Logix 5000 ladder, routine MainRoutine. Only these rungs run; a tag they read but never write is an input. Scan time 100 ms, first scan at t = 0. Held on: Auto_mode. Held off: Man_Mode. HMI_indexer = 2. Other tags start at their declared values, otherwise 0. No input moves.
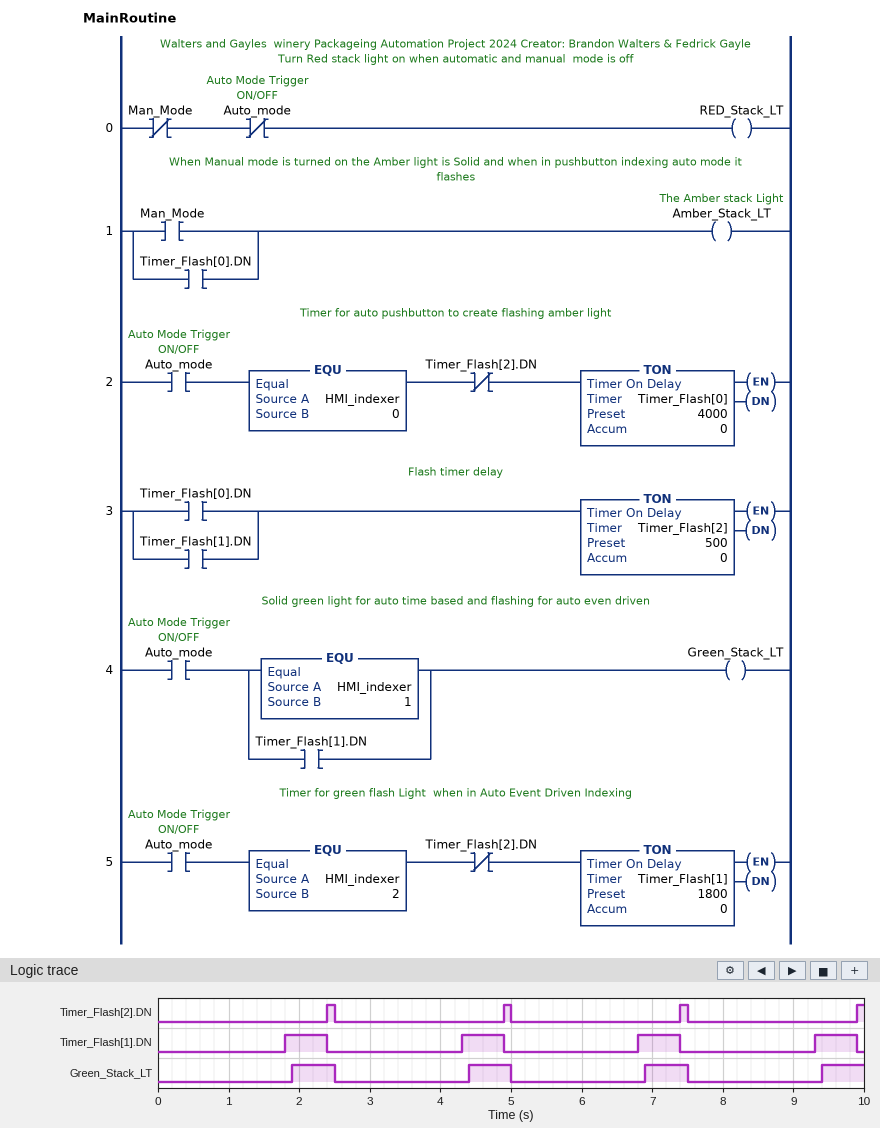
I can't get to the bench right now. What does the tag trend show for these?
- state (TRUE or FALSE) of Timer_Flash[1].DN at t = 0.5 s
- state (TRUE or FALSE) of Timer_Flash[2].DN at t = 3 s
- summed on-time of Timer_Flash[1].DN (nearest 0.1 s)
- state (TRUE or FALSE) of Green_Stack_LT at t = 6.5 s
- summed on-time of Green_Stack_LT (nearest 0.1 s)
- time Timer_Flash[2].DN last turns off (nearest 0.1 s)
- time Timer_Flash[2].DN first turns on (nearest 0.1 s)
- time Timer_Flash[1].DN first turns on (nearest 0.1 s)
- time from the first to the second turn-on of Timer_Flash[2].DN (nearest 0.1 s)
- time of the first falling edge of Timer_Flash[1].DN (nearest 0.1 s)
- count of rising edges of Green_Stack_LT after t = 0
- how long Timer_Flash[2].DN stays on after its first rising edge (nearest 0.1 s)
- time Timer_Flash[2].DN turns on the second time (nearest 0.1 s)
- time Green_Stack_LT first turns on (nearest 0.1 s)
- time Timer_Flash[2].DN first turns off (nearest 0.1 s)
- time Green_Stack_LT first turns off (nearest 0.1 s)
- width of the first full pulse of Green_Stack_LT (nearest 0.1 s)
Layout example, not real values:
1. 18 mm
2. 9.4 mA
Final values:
1. FALSE
2. FALSE
3. 2.4 s
4. FALSE
5. 2.4 s
6. 7.5 s
7. 2.4 s
8. 1.8 s
9. 2.5 s
10. 2.4 s
11. 4
12. 0.1 s
13. 4.9 s
14. 1.9 s
15. 2.5 s
16. 2.5 s
17. 0.6 s
